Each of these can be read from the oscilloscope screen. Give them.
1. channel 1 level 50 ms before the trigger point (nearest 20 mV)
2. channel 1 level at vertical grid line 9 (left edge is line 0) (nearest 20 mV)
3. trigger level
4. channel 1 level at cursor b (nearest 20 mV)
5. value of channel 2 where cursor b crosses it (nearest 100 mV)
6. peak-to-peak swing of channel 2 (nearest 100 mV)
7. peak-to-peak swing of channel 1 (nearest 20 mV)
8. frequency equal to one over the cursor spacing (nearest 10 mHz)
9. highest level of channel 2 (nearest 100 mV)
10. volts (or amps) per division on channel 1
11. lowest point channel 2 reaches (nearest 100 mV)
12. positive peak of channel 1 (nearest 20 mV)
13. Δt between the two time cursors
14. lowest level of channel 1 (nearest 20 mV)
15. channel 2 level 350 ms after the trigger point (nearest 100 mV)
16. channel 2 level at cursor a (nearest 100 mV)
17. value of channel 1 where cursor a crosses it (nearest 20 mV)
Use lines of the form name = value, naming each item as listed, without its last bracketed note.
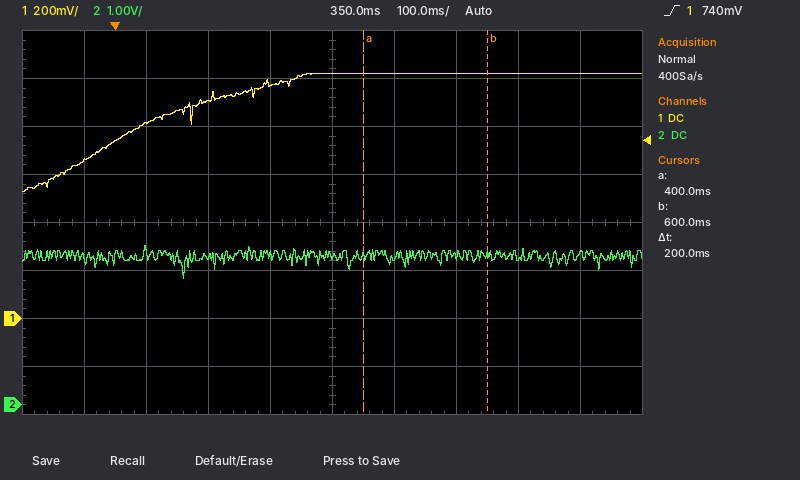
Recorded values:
channel 1 level 50 ms before the trigger point = 660 mV
channel 1 level at vertical grid line 9 (left edge is line 0) = 1.02 V
trigger level = 740 mV
channel 1 level at cursor b = 1.02 V
value of channel 2 where cursor b crosses it = 3.1 V
peak-to-peak swing of channel 2 = 700 mV
peak-to-peak swing of channel 1 = 500 mV
frequency equal to one over the cursor spacing = 5.00 Hz
highest level of channel 2 = 3.3 V
volts (or amps) per division on channel 1 = 200 mV
lowest point channel 2 reaches = 2.6 V
positive peak of channel 1 = 1.02 V
Δt between the two time cursors = 200 ms
lowest level of channel 1 = 520 mV
channel 2 level 350 ms after the trigger point = 3.1 V
channel 2 level at cursor a = 3.1 V
value of channel 1 where cursor a crosses it = 1.02 V
